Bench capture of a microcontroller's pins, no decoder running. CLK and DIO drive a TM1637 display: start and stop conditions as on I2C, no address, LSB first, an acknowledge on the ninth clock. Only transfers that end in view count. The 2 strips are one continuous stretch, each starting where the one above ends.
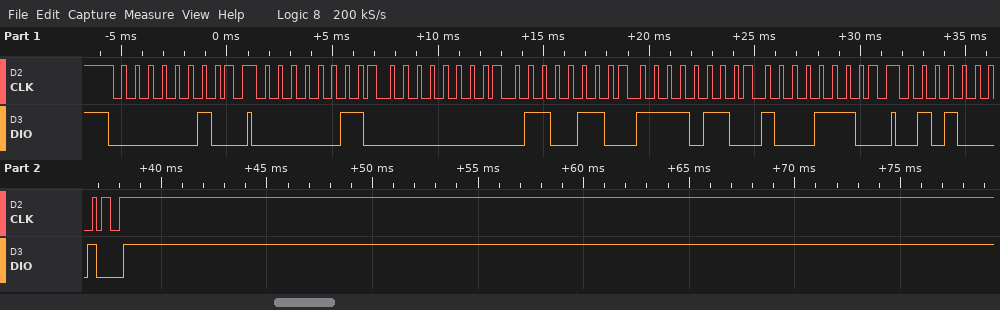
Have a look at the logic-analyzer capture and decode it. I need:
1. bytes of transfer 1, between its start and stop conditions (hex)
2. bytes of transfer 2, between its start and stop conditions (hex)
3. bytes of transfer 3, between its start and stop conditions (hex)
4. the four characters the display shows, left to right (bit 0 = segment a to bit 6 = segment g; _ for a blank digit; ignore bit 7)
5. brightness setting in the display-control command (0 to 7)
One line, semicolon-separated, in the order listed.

40; C0 00 66 6F 71; 8A; _49F; 2
